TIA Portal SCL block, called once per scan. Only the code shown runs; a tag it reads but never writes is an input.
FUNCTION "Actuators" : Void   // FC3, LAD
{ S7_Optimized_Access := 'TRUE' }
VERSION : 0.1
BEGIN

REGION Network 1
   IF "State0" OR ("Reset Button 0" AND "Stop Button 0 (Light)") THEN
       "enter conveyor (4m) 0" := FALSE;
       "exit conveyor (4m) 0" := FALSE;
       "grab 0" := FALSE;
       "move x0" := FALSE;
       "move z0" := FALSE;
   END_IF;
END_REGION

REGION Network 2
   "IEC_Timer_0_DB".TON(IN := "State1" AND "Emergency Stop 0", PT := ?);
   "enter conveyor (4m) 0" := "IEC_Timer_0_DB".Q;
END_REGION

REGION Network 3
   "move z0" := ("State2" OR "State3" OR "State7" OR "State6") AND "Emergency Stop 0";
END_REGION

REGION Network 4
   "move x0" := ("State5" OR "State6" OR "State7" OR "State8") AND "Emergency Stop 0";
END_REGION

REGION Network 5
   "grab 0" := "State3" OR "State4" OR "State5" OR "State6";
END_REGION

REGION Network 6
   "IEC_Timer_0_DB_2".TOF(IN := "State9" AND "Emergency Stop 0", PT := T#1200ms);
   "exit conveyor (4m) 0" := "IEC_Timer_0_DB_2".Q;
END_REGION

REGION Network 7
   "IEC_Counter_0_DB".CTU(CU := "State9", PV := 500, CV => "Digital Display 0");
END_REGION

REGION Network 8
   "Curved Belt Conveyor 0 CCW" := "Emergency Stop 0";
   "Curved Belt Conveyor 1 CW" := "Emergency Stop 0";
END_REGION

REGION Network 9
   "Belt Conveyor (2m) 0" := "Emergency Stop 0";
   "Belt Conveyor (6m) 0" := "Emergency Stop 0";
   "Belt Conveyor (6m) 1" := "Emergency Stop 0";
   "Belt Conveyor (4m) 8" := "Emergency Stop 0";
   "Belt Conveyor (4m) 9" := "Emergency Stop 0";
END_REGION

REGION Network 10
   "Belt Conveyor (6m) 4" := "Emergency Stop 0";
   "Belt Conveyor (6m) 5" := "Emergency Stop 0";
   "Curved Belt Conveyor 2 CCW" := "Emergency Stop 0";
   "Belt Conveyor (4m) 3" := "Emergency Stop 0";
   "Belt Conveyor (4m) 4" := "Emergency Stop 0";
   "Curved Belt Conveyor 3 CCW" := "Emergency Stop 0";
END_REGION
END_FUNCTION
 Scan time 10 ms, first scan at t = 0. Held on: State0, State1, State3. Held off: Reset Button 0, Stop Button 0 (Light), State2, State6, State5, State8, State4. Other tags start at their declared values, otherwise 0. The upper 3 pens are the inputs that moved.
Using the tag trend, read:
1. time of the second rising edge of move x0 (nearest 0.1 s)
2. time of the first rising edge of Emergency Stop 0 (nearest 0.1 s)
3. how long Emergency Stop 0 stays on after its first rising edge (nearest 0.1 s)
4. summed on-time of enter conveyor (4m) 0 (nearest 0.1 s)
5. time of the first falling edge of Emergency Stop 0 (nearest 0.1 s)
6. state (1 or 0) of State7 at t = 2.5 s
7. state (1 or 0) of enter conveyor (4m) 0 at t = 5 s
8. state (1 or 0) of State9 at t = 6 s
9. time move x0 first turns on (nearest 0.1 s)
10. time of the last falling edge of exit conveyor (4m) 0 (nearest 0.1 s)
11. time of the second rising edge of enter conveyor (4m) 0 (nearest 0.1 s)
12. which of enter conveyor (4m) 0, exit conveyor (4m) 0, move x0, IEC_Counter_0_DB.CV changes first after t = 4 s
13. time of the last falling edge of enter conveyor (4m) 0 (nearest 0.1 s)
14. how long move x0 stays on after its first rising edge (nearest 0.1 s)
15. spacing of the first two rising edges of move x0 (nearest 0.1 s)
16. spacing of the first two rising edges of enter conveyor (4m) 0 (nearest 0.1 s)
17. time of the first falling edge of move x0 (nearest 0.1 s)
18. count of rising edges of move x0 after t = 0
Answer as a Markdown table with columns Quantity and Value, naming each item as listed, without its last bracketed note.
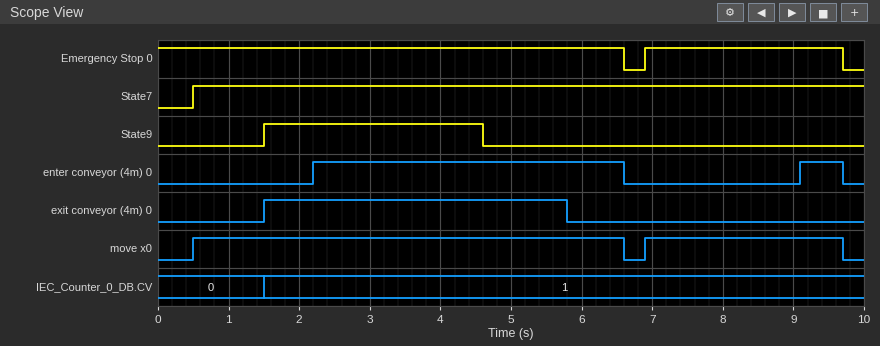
| Quantity | Value |
|---|---|
| time of the second rising edge of move x0 | 6.9 s |
| time of the first rising edge of Emergency Stop 0 | 6.9 s |
| how long Emergency Stop 0 stays on after its first rising edge | 2.8 s |
| summed on-time of enter conveyor (4m) 0 | 5.0 s |
| time of the first falling edge of Emergency Stop 0 | 6.6 s |
| state (1 or 0) of State7 at t = 2.5 s | 1 |
| state (1 or 0) of enter conveyor (4m) 0 at t = 5 s | 1 |
| state (1 or 0) of State9 at t = 6 s | 0 |
| time move x0 first turns on | 0.5 s |
| time of the last falling edge of exit conveyor (4m) 0 | 5.8 s |
| time of the second rising edge of enter conveyor (4m) 0 | 9.1 s |
| which of enter conveyor (4m) 0, exit conveyor (4m) 0, move x0, IEC_Counter_0_DB.CV changes first after t = 4 s | exit conveyor (4m) 0 |
| time of the last falling edge of enter conveyor (4m) 0 | 9.7 s |
| how long move x0 stays on after its first rising edge | 6.1 s |
| spacing of the first two rising edges of move x0 | 6.4 s |
| spacing of the first two rising edges of enter conveyor (4m) 0 | 6.9 s |
| time of the first falling edge of move x0 | 6.6 s |
| count of rising edges of move x0 after t = 0 | 2 |
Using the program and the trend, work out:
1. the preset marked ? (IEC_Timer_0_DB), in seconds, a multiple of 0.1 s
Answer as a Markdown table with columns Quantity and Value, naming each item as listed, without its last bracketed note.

| Quantity | Value |
|---|---|
| the preset marked ? (IEC_Timer_0_DB), in seconds, a multiple of 0.1 s | 2.2 s |
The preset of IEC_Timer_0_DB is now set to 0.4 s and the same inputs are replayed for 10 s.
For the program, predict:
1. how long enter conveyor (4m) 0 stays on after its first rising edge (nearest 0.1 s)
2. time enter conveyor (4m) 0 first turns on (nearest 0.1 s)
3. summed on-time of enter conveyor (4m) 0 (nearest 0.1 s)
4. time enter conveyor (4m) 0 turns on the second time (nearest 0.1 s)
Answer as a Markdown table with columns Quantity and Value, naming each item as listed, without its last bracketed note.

| Quantity | Value |
|---|---|
| how long enter conveyor (4m) 0 stays on after its first rising edge | 6.2 s |
| time enter conveyor (4m) 0 first turns on | 0.4 s |
| summed on-time of enter conveyor (4m) 0 | 8.6 s |
| time enter conveyor (4m) 0 turns on the second time | 7.3 s |
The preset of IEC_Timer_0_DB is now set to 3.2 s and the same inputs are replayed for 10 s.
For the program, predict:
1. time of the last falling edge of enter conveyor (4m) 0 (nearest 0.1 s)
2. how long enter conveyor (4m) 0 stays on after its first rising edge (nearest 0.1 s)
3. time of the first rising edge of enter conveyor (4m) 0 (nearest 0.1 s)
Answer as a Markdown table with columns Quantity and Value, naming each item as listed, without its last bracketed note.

| Quantity | Value |
|---|---|
| time of the last falling edge of enter conveyor (4m) 0 | 6.6 s |
| how long enter conveyor (4m) 0 stays on after its first rising edge | 3.4 s |
| time of the first rising edge of enter conveyor (4m) 0 | 3.2 s |
